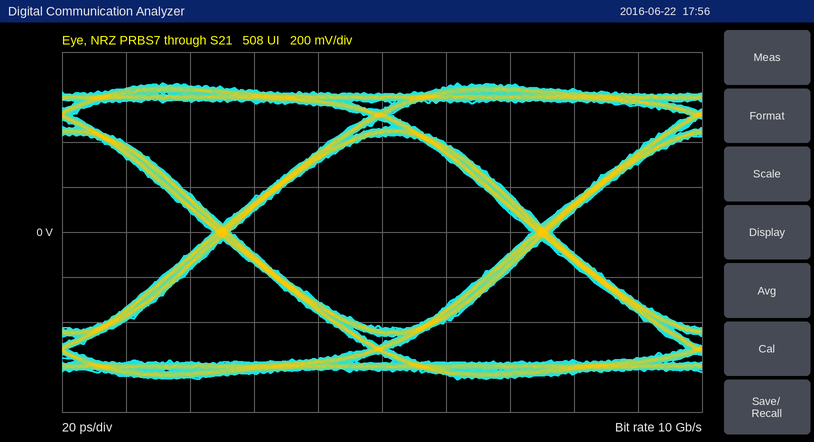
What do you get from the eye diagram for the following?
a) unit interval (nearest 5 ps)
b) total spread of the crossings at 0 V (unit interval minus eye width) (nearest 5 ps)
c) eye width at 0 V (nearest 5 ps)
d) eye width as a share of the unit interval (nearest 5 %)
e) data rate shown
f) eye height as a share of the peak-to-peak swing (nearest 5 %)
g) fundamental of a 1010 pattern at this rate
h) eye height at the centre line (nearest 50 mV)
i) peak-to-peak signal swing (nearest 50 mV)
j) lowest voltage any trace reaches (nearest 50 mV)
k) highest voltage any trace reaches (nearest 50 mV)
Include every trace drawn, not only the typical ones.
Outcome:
100 ps
5 ps
95 ps
95 %
10 Gb/s
65 %
5 GHz
850 mV
1.30 V
-650 mV
650 mV
